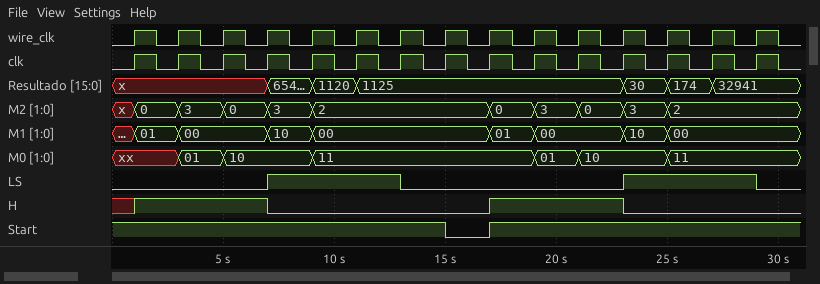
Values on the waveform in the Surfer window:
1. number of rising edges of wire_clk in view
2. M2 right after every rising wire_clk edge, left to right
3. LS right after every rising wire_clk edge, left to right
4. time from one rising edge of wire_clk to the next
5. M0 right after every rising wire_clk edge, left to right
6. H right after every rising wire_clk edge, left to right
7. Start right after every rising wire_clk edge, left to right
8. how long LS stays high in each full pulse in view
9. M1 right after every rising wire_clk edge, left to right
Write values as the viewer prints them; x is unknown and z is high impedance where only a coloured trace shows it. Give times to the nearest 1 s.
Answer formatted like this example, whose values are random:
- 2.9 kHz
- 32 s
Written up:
- 15
- 0, 3, 0, 3, 2, 2, 2, 2, 0, 3, 0, 3, 2, 2, 2
- 0 0 0 1 1 1 0 0 0 0 0 1 1 1 0
- 2 s
- xx, 01, 10, 10, 11, 11, 11, 11, 11, 01, 10, 10, 11, 11, 11
- 1 1 1 0 0 0 0 0 1 1 1 0 0 0 0
- 1 1 1 1 1 1 1 0 1 1 1 1 1 1 1
- 6 s, 6 s
- 01, 00, 00, 10, 00, 00, 00, 00, 01, 00, 00, 10, 00, 00, 00
